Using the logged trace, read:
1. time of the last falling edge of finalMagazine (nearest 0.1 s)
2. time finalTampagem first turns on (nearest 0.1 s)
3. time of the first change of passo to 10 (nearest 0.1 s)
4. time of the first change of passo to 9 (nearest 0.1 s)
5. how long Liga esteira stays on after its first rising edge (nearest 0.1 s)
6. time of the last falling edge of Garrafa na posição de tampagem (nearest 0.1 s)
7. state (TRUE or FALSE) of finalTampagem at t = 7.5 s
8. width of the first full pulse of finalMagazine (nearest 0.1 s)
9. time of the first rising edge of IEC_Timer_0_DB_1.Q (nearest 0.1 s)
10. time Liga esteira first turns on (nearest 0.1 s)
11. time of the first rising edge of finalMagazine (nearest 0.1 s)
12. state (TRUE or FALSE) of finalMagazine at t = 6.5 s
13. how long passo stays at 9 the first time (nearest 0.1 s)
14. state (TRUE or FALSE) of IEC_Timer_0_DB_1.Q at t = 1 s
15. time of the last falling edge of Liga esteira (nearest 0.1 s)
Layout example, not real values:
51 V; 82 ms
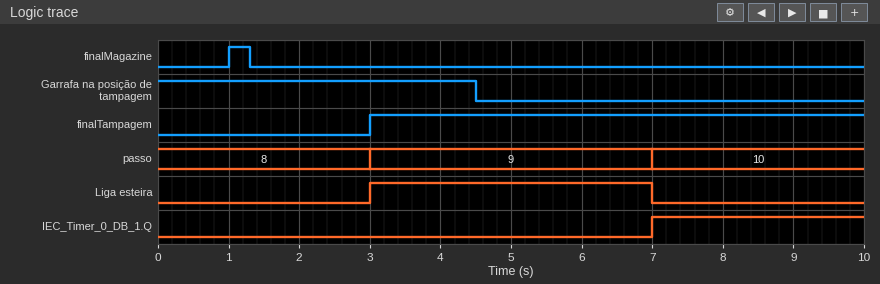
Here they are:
1.3 s; 3.0 s; 7.0 s; 3.0 s; 4.0 s; 4.5 s; TRUE; 0.3 s; 7.0 s; 3.0 s; 1.0 s; FALSE; 4.0 s; FALSE; 7.0 s
